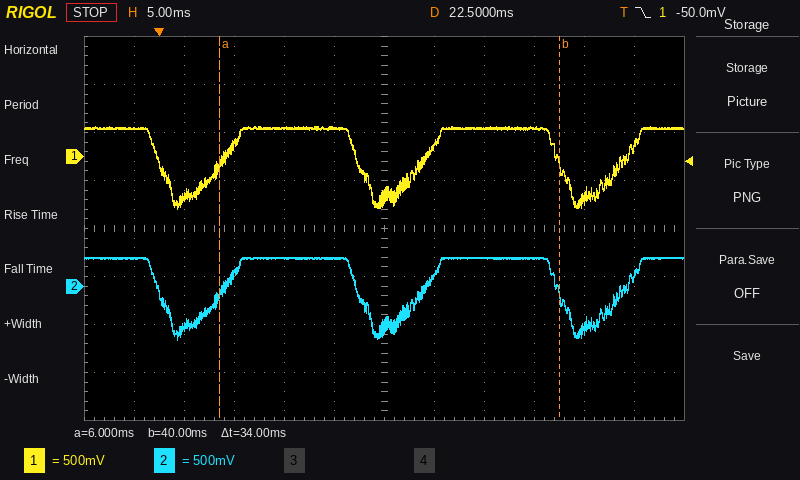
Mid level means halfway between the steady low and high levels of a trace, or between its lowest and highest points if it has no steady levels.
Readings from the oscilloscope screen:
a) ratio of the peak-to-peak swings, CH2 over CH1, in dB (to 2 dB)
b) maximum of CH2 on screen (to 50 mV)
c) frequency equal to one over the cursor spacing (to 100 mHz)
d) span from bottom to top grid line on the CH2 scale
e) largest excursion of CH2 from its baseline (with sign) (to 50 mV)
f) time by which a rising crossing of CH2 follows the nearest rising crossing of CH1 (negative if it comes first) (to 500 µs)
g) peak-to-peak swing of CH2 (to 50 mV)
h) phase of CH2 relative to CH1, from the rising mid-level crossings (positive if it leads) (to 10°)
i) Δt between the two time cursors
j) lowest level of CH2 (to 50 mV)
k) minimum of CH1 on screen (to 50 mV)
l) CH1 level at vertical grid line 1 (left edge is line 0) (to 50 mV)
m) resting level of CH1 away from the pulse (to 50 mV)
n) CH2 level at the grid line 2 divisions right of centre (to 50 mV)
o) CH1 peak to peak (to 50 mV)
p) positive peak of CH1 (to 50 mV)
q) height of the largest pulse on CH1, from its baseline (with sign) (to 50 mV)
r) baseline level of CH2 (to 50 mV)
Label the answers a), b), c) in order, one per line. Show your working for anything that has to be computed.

a) 20 log10(850 mV / 850 mV) ≈ 0 dB
b) 300 mV
c) 1 / 34 ms ≈ 29.4 Hz
d) 4 V
e) -550 mV − (300 mV) = -850 mV
f) 0.0 ms
g) 300 mV − (-550 mV) = 850 mV
h) 0°
i) 34 ms
j) -550 mV
k) -550 mV
l) 300 mV
m) 300 mV
n) 300 mV
o) 300 mV − (-550 mV) = 850 mV
p) 300 mV
q) -550 mV − (300 mV) = -850 mV
r) 300 mV
